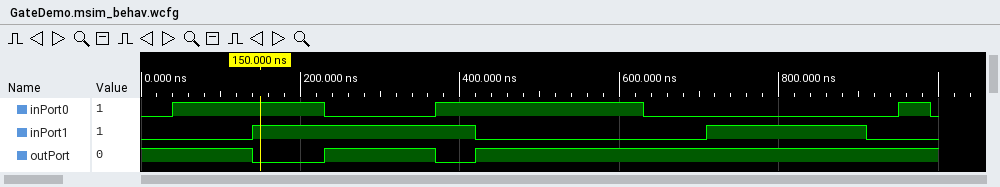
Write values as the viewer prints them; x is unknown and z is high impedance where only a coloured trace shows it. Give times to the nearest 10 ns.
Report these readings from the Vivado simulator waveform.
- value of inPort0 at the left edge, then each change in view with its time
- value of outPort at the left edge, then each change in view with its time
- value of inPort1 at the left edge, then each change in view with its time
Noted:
0, 1 at 40 ns, 0 at 230 ns, 1 at 370 ns, 0 at 630 ns, 1 at 950 ns, 0 at 990 ns
1, 0 at 140 ns, 1 at 230 ns, 0 at 370 ns, 1 at 420 ns
0, 1 at 140 ns, 0 at 420 ns, 1 at 710 ns, 0 at 910 ns
